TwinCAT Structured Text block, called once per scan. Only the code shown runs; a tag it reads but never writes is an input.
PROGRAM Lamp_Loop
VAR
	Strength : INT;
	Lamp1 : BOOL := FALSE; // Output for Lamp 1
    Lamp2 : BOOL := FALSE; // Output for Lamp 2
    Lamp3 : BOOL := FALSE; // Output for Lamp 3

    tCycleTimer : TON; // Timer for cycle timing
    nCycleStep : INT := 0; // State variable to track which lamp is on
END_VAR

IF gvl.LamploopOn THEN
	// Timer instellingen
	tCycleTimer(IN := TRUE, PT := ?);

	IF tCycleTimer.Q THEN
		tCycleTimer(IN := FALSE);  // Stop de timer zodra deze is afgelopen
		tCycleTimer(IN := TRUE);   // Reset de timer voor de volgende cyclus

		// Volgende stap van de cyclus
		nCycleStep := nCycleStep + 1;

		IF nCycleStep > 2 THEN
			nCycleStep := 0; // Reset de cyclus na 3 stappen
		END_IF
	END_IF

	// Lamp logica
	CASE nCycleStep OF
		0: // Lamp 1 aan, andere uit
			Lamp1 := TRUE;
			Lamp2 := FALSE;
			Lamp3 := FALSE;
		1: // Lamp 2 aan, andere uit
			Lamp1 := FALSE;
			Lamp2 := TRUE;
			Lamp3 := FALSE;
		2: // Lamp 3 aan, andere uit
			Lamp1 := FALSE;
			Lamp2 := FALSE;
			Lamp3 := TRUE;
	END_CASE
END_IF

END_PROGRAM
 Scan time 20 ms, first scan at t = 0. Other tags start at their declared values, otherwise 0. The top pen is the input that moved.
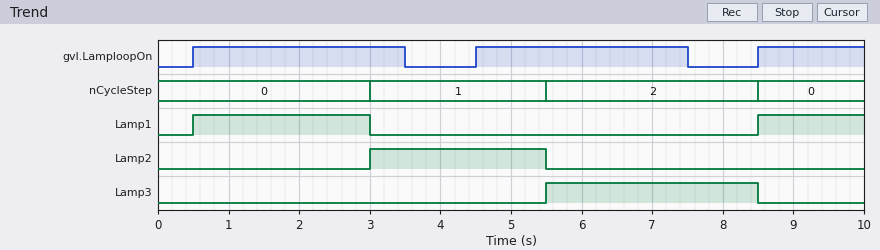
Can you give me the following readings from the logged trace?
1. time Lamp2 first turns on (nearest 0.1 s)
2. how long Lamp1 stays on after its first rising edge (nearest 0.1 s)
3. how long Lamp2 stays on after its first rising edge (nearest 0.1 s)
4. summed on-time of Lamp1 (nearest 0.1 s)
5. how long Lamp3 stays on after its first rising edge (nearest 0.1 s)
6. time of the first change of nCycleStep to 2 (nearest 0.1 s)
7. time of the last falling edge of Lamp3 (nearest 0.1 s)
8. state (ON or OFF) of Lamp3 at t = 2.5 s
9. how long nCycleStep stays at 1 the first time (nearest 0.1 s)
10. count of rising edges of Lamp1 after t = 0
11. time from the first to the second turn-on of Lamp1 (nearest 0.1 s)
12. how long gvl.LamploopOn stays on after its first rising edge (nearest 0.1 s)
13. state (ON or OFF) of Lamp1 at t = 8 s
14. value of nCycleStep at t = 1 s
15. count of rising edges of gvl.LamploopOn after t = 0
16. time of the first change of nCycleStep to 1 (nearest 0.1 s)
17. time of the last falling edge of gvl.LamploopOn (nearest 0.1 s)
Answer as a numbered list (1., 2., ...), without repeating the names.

1. 3.0 s
2. 2.5 s
3. 2.5 s
4. 4.0 s
5. 3.0 s
6. 5.5 s
7. 8.5 s
8. OFF
9. 2.5 s
10. 2
11. 8.0 s
12. 3.0 s
13. OFF
14. 0
15. 3
16. 3.0 s
17. 7.5 s
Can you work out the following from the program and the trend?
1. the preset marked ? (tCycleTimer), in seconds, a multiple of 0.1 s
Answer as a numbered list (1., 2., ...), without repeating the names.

1. 2.5 s
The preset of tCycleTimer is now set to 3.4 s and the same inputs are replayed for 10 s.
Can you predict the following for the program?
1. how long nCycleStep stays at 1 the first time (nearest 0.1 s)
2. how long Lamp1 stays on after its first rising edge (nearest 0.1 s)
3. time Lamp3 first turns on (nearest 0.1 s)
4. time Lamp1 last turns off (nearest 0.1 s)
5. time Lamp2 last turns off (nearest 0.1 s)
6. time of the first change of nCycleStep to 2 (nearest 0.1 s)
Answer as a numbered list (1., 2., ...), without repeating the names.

1. 4.0 s
2. 4.0 s
3. 8.5 s
4. 4.5 s
5. 8.5 s
6. 8.5 s
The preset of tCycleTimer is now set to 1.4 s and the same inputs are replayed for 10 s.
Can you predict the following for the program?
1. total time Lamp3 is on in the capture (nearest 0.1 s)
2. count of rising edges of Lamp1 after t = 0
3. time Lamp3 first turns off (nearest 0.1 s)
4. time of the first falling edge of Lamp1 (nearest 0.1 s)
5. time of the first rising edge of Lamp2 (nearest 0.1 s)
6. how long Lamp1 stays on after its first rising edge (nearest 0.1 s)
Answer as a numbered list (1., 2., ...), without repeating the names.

1. 2.8 s
2. 3
3. 4.7 s
4. 1.9 s
5. 1.9 s
6. 1.4 s
